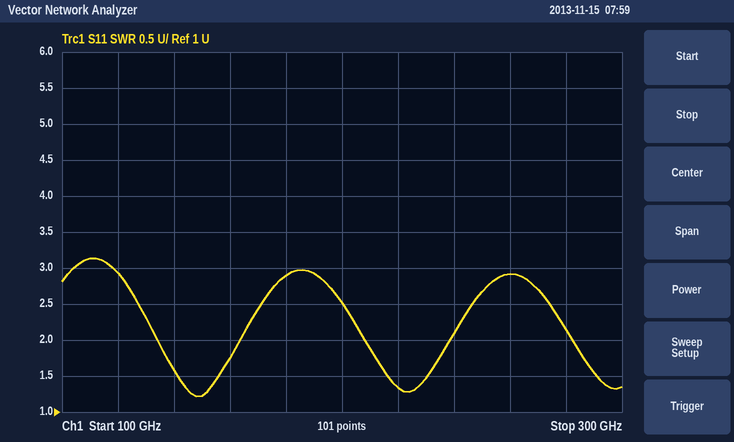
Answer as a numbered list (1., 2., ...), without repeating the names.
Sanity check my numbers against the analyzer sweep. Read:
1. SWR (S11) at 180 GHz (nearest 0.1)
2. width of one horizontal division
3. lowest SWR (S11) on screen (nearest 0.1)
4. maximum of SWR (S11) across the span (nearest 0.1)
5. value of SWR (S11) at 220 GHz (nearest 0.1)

1. 2.9
2. 20 GHz
3. 1.2
4. 3.1
5. 1.3
